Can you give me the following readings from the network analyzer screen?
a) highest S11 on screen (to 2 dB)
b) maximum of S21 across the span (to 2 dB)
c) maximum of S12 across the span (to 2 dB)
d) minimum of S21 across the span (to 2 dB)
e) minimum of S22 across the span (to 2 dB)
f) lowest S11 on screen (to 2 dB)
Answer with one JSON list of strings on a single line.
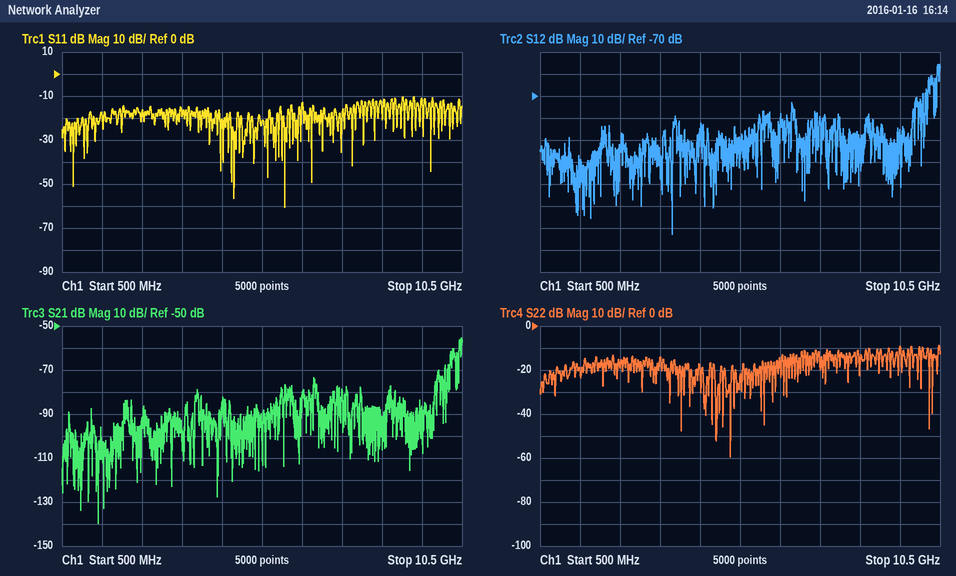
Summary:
["-10 dB", "-56 dB", "-56 dB", "-140 dB", "-60 dB", "-60 dB"]
